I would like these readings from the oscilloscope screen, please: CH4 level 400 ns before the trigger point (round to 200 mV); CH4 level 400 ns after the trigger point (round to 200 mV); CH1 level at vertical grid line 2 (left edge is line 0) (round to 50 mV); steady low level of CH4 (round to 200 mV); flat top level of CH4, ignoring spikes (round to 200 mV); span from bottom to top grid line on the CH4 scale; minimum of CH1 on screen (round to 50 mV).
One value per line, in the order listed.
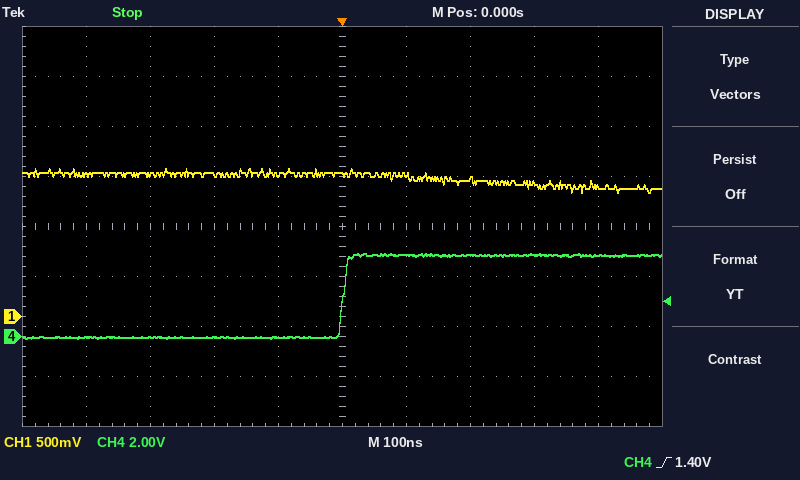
0.0 V
3.2 V
1.40 V
0.0 V
3.2 V
16 V
1.25 V
